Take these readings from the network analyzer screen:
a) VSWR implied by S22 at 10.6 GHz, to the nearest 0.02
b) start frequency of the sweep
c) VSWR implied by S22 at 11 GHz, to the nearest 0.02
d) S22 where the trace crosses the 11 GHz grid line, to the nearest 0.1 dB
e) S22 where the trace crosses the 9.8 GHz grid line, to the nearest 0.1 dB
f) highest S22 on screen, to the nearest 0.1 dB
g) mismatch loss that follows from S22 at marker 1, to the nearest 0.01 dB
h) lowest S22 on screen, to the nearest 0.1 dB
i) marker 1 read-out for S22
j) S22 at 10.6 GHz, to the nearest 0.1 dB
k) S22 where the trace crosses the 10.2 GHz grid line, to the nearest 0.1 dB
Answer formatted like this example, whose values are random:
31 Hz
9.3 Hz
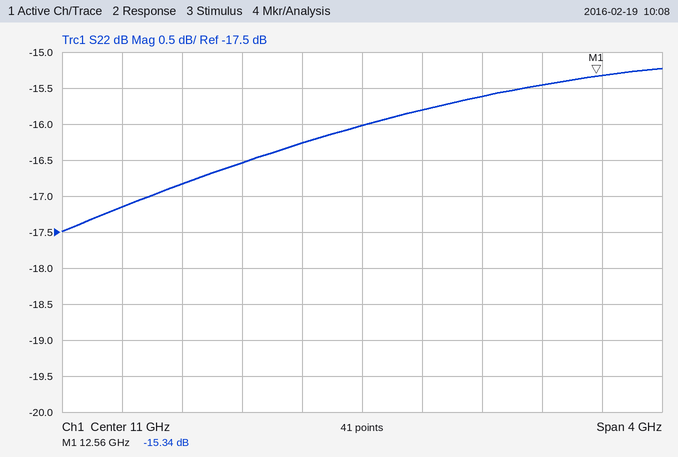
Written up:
1.36
9 GHz
1.38
-16.0 dB
-16.8 dB
-15.2 dB
0.13 dB
-17.5 dB
-15.34 dB
-16.3 dB
-16.5 dB
